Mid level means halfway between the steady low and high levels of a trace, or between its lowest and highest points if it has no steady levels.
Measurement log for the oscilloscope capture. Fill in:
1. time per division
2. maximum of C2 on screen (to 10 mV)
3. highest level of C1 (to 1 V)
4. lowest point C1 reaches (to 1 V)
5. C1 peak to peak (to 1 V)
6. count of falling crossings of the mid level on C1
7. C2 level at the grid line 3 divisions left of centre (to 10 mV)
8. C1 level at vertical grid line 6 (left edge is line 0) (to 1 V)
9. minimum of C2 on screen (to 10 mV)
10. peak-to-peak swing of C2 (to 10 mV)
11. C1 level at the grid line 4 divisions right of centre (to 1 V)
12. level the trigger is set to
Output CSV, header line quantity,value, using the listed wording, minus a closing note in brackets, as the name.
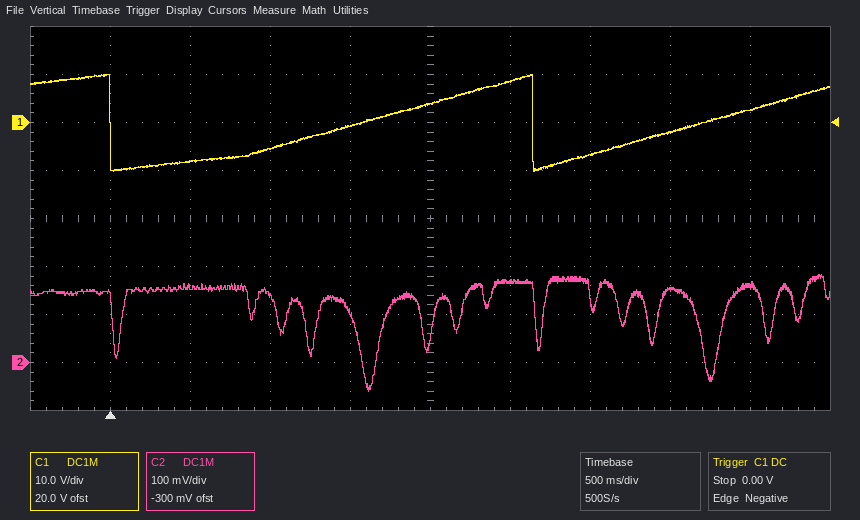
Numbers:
quantity,value
time per division,500 ms
maximum of C2 on screen,180 mV
highest level of C1,10 V
lowest point C1 reaches,-10 V
C1 peak to peak,20 V
count of falling crossings of the mid level on C1,2
C2 level at the grid line 3 divisions left of centre,160 mV
C1 level at vertical grid line 6 (left edge is line 0),9 V
minimum of C2 on screen,-60 mV
peak-to-peak swing of C2,240 mV
C1 level at the grid line 4 divisions right of centre,3 V
level the trigger is set to,0.00 V
